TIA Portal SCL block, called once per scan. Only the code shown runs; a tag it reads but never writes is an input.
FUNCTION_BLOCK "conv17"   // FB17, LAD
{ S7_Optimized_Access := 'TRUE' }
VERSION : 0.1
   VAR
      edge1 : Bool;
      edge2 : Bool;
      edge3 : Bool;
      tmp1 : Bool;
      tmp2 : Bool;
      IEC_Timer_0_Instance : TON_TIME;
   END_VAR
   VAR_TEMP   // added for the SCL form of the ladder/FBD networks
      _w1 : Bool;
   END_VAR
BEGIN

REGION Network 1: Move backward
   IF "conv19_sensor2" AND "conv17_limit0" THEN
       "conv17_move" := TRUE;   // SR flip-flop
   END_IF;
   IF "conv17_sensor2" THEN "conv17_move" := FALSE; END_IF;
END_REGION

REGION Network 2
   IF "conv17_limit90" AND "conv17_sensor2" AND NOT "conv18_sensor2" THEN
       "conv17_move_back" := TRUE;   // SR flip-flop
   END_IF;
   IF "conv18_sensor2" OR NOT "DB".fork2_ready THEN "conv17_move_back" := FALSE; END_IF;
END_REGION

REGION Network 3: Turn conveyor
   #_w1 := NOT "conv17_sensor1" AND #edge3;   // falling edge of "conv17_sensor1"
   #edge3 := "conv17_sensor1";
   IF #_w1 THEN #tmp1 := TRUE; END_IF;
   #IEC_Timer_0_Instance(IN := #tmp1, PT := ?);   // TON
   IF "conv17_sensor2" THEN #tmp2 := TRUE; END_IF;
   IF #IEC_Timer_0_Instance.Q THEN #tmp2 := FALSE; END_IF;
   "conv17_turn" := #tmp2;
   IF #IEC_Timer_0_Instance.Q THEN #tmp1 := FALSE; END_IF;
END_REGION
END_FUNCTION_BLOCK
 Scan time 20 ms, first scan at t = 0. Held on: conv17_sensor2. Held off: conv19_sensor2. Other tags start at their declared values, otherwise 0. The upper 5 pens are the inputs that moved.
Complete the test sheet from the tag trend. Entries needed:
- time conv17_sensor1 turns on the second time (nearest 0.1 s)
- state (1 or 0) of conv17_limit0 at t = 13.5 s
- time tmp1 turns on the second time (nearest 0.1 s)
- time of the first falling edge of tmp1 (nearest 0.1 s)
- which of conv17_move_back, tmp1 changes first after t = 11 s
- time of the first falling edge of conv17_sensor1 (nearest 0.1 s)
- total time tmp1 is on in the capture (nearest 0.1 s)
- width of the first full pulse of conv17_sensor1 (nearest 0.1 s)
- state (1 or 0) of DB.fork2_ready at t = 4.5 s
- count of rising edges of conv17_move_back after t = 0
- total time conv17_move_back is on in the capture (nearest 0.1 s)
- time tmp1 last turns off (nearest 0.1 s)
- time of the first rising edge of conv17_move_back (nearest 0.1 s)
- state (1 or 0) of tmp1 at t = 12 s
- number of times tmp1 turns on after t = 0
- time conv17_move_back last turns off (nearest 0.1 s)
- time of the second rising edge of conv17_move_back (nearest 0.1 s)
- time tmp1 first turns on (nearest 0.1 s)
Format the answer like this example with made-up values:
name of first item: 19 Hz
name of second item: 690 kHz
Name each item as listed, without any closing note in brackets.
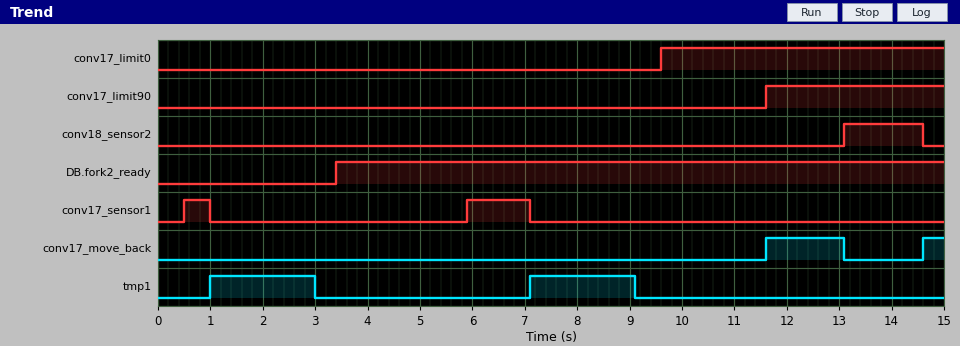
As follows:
time conv17_sensor1 turns on the second time: 5.9 s
state (1 or 0) of conv17_limit0 at t = 13.5 s: 1
time tmp1 turns on the second time: 7.1 s
time of the first falling edge of tmp1: 3.0 s
which of conv17_move_back, tmp1 changes first after t = 11 s: conv17_move_back
time of the first falling edge of conv17_sensor1: 1.0 s
total time tmp1 is on in the capture: 4.0 s
width of the first full pulse of conv17_sensor1: 0.5 s
state (1 or 0) of DB.fork2_ready at t = 4.5 s: 1
count of rising edges of conv17_move_back after t = 0: 2
total time conv17_move_back is on in the capture: 1.9 s
time tmp1 last turns off: 9.1 s
time of the first rising edge of conv17_move_back: 11.6 s
state (1 or 0) of tmp1 at t = 12 s: 0
number of times tmp1 turns on after t = 0: 2
time conv17_move_back last turns off: 13.1 s
time of the second rising edge of conv17_move_back: 14.6 s
time tmp1 first turns on: 1.0 s
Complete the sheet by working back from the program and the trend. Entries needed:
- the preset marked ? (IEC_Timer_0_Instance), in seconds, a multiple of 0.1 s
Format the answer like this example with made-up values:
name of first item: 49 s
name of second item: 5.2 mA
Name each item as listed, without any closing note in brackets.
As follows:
the preset marked ? (IEC_Timer_0_Instance), in seconds, a multiple of 0.1 s: 2.0 s
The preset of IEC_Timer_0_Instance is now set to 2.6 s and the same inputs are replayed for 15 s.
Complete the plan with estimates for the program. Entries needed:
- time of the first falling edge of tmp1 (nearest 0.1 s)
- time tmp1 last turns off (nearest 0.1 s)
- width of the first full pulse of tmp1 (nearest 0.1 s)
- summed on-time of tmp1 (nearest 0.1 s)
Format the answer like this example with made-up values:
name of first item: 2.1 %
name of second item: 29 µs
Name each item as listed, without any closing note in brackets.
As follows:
time of the first falling edge of tmp1: 3.6 s
time tmp1 last turns off: 9.7 s
width of the first full pulse of tmp1: 2.6 s
summed on-time of tmp1: 5.2 s
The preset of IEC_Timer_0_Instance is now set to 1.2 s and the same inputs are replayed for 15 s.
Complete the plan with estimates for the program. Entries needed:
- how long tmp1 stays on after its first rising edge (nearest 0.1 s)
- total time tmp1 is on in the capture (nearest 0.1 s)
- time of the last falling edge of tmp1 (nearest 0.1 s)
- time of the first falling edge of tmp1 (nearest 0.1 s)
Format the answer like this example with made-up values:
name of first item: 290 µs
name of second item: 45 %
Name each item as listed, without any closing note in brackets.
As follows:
how long tmp1 stays on after its first rising edge: 1.2 s
total time tmp1 is on in the capture: 2.4 s
time of the last falling edge of tmp1: 8.3 s
time of the first falling edge of tmp1: 2.2 s
